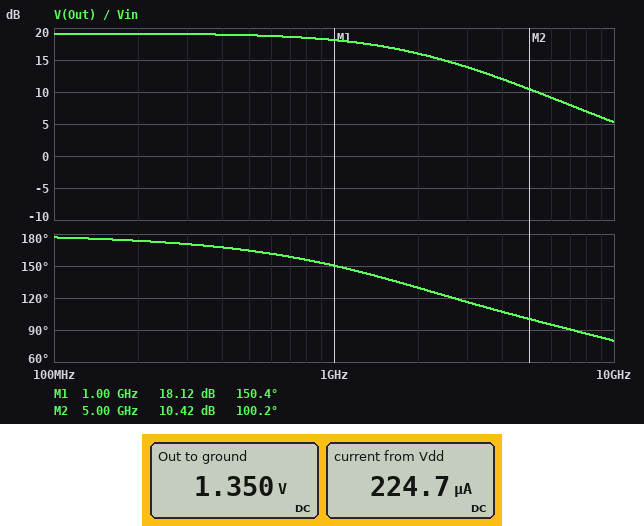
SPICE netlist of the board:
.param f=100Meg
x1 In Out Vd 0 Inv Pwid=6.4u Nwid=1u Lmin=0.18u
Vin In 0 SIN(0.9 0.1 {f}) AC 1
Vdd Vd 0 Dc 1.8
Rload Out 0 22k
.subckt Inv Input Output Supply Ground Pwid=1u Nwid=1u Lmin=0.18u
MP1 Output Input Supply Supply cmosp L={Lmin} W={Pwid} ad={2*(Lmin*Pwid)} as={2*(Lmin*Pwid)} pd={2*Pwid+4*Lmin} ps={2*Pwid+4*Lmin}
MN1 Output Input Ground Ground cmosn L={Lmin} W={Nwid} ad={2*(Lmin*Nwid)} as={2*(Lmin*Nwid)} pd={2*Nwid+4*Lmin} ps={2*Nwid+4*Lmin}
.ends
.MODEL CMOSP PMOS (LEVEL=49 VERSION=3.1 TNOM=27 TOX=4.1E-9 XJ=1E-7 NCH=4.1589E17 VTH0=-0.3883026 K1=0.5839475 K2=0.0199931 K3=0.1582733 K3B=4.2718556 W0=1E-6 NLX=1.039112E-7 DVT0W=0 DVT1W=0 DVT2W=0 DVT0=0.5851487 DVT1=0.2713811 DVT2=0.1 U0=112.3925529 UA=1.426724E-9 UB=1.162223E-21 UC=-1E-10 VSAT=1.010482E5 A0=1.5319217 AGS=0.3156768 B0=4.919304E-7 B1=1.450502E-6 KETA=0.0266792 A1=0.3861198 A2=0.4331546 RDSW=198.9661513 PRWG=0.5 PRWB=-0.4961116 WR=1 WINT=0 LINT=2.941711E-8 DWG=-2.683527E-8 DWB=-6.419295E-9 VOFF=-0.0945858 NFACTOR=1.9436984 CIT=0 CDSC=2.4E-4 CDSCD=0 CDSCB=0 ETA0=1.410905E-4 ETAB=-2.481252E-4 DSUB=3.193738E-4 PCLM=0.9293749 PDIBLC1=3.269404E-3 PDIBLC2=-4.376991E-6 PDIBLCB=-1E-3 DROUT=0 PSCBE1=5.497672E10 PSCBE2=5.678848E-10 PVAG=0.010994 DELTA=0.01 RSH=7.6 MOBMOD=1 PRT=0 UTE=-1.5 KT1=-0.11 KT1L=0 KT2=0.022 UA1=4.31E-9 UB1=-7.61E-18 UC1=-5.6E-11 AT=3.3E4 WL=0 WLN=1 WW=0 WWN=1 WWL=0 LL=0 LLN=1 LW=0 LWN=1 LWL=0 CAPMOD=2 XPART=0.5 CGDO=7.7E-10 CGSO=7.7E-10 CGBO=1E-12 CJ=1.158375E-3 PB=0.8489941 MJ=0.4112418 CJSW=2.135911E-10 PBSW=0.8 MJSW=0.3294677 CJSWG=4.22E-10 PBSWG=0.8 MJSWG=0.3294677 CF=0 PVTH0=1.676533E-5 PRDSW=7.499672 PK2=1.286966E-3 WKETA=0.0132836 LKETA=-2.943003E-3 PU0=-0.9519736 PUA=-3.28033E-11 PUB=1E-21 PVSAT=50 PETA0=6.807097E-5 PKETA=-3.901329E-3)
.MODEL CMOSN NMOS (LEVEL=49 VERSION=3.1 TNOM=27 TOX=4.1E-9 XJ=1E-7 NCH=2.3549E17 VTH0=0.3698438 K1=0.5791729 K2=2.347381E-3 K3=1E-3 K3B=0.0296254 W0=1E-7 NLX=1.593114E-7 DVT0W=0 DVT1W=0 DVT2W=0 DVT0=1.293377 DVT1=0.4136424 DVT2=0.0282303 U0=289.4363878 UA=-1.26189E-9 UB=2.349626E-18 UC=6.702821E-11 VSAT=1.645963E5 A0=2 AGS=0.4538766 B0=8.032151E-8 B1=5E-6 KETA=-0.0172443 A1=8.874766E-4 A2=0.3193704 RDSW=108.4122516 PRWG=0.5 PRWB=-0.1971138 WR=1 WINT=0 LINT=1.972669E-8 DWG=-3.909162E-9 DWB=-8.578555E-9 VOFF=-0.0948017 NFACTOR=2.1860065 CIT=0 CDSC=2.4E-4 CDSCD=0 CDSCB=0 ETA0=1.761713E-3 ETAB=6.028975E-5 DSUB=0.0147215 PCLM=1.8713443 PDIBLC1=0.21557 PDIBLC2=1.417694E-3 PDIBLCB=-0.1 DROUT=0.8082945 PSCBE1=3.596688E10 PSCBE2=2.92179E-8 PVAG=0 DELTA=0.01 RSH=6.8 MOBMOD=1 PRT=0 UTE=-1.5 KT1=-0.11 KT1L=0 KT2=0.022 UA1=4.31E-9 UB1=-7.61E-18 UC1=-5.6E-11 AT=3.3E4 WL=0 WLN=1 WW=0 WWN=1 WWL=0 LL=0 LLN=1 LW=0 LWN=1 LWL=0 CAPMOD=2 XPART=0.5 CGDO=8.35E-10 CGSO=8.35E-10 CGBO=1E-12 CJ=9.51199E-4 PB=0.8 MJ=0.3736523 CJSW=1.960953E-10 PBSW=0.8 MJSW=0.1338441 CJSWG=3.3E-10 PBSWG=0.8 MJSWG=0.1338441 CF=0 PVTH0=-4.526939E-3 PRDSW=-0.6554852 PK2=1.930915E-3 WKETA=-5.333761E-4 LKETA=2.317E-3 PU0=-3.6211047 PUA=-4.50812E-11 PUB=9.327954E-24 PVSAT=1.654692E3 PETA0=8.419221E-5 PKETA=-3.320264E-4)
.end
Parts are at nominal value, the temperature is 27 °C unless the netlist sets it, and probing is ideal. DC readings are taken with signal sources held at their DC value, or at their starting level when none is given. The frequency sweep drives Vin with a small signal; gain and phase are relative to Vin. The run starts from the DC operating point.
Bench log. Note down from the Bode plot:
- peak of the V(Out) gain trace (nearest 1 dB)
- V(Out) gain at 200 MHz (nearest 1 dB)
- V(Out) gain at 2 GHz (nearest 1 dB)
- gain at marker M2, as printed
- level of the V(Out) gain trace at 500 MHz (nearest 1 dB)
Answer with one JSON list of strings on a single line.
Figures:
["19 dB", "19 dB", "16 dB", "10.42 dB", "19 dB"]
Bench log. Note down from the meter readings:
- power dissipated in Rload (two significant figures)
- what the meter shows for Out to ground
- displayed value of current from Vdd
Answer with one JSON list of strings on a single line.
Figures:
["83 µW", "1.350 V", "224.7 µA"]
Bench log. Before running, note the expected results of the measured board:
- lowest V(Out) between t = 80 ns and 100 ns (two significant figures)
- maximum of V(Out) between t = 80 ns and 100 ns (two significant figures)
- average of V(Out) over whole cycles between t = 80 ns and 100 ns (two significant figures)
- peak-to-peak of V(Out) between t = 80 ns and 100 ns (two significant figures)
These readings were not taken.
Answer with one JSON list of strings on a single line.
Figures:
["230 mV", "1.6 V", "1.1 V", "1.4 V"]
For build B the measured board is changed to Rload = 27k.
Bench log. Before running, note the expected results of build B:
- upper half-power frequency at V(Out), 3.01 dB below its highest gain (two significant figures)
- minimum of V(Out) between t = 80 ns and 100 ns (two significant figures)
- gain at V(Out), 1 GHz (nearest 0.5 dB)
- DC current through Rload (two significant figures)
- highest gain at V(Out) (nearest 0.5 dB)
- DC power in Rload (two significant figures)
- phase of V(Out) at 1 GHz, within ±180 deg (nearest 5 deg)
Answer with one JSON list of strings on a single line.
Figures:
["2.3 GHz", "240 mV", "16.5 dB", "53 µA", "17.5 dB", "75 µW", "155 deg"]
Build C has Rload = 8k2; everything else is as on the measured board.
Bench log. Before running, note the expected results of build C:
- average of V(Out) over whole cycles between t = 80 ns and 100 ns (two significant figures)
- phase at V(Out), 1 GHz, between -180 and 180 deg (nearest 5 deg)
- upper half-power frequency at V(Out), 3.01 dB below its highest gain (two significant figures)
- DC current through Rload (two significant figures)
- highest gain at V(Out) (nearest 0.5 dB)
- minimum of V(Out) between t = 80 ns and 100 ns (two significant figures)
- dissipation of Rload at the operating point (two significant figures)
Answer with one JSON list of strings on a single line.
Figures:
["810 mV", "155 deg", "2.3 GHz", "97 µA", "18.5 dB", "200 mV", "77 µW"]
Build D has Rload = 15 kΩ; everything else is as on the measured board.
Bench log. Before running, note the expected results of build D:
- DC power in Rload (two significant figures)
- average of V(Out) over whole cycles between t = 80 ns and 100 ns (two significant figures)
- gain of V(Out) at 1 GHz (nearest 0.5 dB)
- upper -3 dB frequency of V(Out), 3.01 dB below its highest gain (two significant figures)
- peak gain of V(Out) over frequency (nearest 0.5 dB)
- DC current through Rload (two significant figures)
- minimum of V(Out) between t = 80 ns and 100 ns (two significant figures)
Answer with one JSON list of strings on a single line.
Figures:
["89 µW", "990 mV", "19.5 dB", "1.7 GHz", "20.5 dB", "77 µA", "220 mV"]
